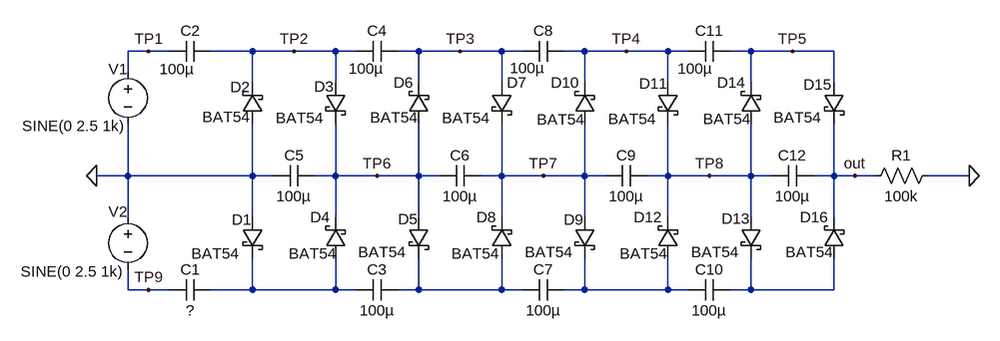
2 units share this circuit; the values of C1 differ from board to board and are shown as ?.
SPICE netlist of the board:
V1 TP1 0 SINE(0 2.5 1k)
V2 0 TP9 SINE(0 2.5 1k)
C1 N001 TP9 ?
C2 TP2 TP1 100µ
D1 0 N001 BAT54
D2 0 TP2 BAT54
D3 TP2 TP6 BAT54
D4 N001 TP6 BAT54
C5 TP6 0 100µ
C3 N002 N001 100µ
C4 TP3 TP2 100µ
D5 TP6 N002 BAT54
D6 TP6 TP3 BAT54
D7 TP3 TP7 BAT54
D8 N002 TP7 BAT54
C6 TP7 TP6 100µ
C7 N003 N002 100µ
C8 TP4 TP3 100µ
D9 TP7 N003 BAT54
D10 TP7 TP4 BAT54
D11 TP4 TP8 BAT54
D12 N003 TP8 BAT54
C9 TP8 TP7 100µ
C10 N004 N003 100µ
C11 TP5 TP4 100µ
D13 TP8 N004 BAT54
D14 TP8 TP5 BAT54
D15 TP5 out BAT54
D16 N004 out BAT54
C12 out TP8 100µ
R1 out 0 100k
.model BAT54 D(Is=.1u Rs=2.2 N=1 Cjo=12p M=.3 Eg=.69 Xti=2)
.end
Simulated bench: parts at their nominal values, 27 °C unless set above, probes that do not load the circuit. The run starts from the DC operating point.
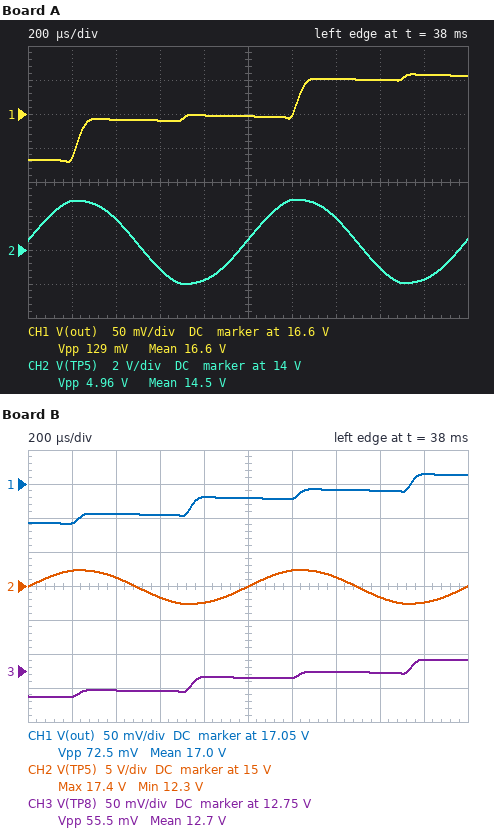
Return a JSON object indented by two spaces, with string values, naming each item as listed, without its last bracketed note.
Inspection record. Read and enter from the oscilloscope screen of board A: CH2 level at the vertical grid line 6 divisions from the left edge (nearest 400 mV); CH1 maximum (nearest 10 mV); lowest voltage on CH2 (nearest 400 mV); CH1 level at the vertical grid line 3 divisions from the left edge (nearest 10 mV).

{
  "CH2 level at the vertical grid line 6 divisions from the left edge": "16.8 V",
  "CH1 maximum": "16.66 V",
  "lowest voltage on CH2": "12.0 V",
  "CH1 level at the vertical grid line 3 divisions from the left edge": "16.59 V"
}
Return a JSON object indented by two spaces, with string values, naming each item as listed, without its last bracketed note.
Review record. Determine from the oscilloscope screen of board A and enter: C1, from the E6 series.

{
  "C1, from the E6 series": "47 µF"
}
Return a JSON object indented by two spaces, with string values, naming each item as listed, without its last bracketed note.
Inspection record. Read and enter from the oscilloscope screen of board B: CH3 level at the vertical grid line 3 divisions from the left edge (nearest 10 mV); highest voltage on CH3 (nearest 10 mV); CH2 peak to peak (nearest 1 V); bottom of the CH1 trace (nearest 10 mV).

{
  "CH3 level at the vertical grid line 3 divisions from the left edge": "12.72 V",
  "highest voltage on CH3": "12.77 V",
  "CH2 peak to peak": "5 V",
  "bottom of the CH1 trace": "16.99 V"
}
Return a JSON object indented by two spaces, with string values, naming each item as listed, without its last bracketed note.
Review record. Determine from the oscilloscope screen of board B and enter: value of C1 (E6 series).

{
  "value of C1": "220 µF"
}
